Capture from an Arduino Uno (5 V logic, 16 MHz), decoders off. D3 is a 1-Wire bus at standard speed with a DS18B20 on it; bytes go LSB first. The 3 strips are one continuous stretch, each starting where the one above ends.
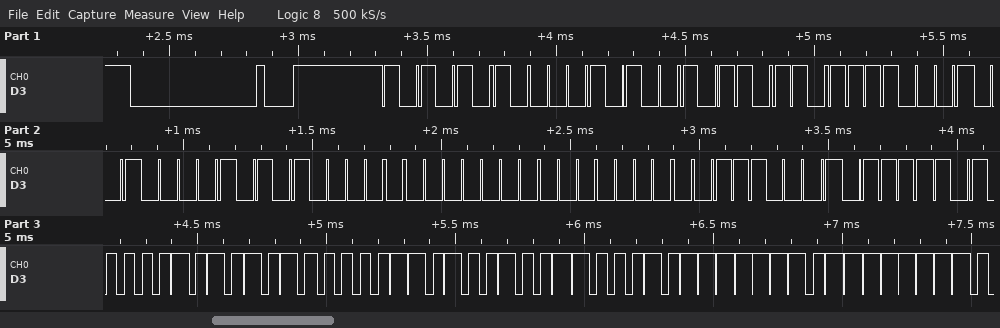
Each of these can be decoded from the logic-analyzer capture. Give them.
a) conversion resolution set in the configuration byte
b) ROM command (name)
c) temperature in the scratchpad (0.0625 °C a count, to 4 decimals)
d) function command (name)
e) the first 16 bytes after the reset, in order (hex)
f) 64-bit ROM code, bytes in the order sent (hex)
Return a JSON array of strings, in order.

["12 bits", "Match ROM", "85.0000 °C", "Read Scratchpad", "55 28 6D 8F 84 0A 00 00 8E BE 50 05 4B 46 7F FF", "28 6D 8F 84 0A 00 00 8E"]
